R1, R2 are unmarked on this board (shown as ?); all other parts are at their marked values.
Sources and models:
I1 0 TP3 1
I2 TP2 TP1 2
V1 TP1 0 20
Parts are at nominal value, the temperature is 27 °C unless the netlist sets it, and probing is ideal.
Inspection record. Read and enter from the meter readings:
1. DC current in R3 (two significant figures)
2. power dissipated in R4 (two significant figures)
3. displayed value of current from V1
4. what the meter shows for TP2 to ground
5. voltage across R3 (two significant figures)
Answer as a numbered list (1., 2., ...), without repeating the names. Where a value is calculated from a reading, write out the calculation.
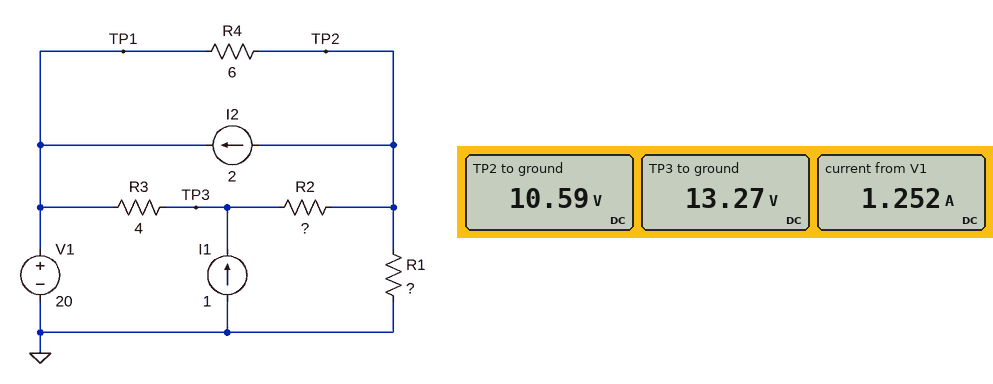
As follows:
1. (20 V - 13.27 V) / 4 Ω = 1.7 A
2. (20 V - 10.59 V)^2 / 6 Ω = 15 W
3. 1.252 A
4. 10.59 V
5. 20 V - 13.27 V = 6.7 V
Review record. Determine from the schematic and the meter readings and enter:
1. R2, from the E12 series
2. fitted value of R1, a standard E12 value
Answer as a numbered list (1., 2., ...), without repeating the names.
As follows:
1. 1 Ω
2. 4.7 Ω
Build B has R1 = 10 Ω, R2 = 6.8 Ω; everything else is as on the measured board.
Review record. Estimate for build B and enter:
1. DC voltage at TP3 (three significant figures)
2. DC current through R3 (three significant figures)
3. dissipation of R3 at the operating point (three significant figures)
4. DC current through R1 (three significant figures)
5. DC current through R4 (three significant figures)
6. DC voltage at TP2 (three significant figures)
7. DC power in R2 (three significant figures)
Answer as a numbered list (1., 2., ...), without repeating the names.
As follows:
1. 18.8 V
2. 306 mA
3. 374 mW
4. 990 mA
5. 1.68 A
6. 9.90 V
7. 11.6 W
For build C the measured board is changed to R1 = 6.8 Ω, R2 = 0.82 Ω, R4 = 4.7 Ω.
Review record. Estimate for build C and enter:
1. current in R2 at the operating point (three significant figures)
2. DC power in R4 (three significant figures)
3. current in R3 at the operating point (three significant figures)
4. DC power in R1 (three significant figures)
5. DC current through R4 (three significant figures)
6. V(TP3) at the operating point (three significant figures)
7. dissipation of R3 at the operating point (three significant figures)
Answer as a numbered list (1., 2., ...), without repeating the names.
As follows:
1. 2.33 A
2. 11.2 W
3. 1.33 A
4. 23.9 W
5. 1.54 A
6. 14.7 V
7. 7.11 W
